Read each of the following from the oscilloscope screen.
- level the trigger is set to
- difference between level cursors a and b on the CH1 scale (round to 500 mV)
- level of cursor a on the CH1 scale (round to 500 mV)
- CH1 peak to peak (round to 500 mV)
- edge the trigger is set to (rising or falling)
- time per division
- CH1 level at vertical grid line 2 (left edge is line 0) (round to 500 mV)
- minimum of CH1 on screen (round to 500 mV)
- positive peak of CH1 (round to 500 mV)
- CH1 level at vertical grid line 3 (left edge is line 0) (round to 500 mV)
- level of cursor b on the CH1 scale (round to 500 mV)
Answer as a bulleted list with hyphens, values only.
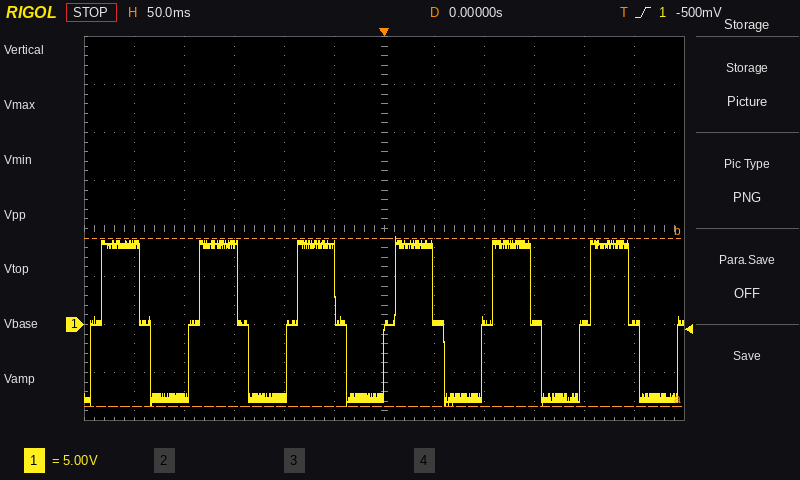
- -500 mV
- 17.5 V
- -8.5 V
- 17.5 V
- rising
- 50 ms
- -7.5 V
- -8.5 V
- 9.0 V
- 8.5 V
- 9.0 V
